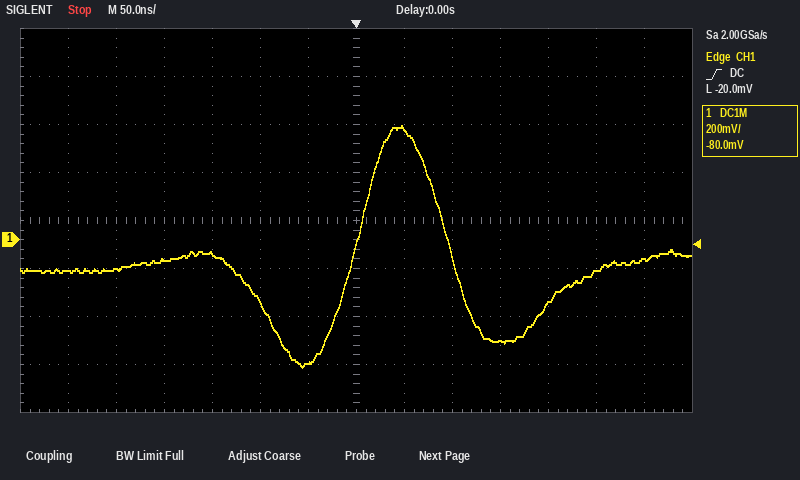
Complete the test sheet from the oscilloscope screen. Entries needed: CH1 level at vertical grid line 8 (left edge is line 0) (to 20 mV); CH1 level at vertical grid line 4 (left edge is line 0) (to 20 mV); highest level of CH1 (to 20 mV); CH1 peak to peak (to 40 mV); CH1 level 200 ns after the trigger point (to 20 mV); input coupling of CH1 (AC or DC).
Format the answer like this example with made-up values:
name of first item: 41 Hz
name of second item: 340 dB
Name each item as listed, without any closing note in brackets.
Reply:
CH1 level at vertical grid line 8 (left edge is line 0): 460 mV
CH1 level at vertical grid line 4 (left edge is line 0): -60 mV
highest level of CH1: 480 mV
CH1 peak to peak: 1.00 V
CH1 level 200 ns after the trigger point: -260 mV
input coupling of CH1: DC
